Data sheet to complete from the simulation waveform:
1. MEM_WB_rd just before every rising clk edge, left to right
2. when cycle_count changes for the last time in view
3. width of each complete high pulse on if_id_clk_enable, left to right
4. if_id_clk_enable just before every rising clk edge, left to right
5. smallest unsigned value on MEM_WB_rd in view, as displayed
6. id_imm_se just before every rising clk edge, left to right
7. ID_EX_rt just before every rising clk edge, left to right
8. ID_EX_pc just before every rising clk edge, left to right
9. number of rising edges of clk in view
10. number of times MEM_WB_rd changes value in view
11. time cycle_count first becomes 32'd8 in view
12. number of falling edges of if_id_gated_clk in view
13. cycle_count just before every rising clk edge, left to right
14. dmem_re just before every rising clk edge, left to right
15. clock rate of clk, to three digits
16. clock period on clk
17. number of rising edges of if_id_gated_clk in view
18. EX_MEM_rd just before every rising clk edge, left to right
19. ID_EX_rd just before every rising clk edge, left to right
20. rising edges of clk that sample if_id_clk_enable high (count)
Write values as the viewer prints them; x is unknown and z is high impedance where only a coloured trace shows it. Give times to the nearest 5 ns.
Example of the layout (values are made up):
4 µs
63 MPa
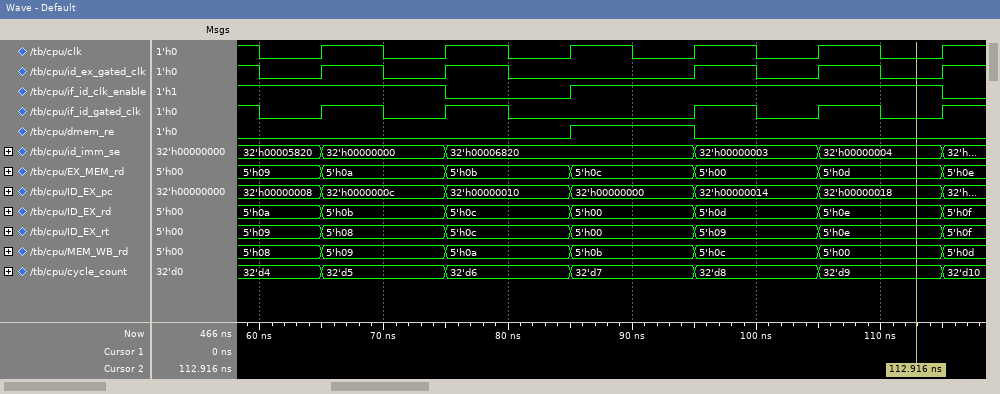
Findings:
5'h08, 5'h09, 5'h0a, 5'h0b, 5'h0c, 5'h00
115 ns
30 ns
1 1 0 1 1 1
5'h00
32'h00005820, 32'h00000000, 32'h00006820, 32'h00006820, 32'h00000003, 32'h00000004
5'h09, 5'h08, 5'h0c, 5'h00, 5'h09, 5'h0e
32'h00000008, 32'h0000000c, 32'h00000010, 32'h00000000, 32'h00000014, 32'h00000018
6
6
95 ns
5
32'd4, 32'd5, 32'd6, 32'd7, 32'd8, 32'd9
0 0 0 1 0 0
100 MHz
10 ns
5
5'h09, 5'h0a, 5'h0b, 5'h0c, 5'h00, 5'h0d
5'h0a, 5'h0b, 5'h0c, 5'h00, 5'h0d, 5'h0e
5
